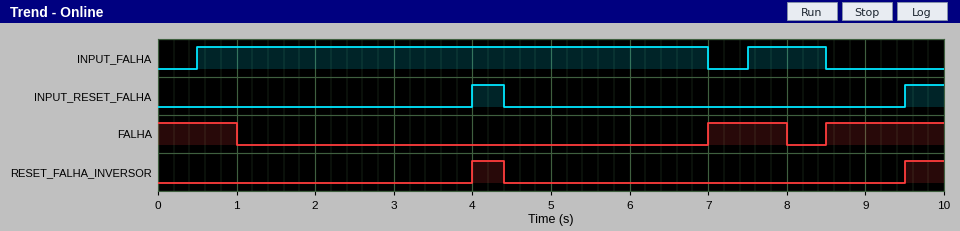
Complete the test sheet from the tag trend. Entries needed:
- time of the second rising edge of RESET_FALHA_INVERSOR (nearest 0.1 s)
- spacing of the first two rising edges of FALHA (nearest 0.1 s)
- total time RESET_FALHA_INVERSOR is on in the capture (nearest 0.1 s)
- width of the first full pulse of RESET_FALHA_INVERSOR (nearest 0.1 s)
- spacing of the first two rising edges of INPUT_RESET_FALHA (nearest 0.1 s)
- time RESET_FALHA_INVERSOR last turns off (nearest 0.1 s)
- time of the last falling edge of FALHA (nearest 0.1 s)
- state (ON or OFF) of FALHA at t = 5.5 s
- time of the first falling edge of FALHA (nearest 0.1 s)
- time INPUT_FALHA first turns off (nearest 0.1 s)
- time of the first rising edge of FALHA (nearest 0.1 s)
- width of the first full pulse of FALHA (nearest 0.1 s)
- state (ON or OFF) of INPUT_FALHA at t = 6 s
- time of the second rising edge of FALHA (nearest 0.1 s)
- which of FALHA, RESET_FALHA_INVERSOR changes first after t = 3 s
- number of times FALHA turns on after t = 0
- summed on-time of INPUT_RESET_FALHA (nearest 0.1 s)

9.5 s
1.5 s
0.9 s
0.4 s
5.5 s
4.4 s
8.0 s
OFF
1.0 s
7.0 s
7.0 s
1.0 s
ON
8.5 s
RESET_FALHA_INVERSOR
2
0.9 s
